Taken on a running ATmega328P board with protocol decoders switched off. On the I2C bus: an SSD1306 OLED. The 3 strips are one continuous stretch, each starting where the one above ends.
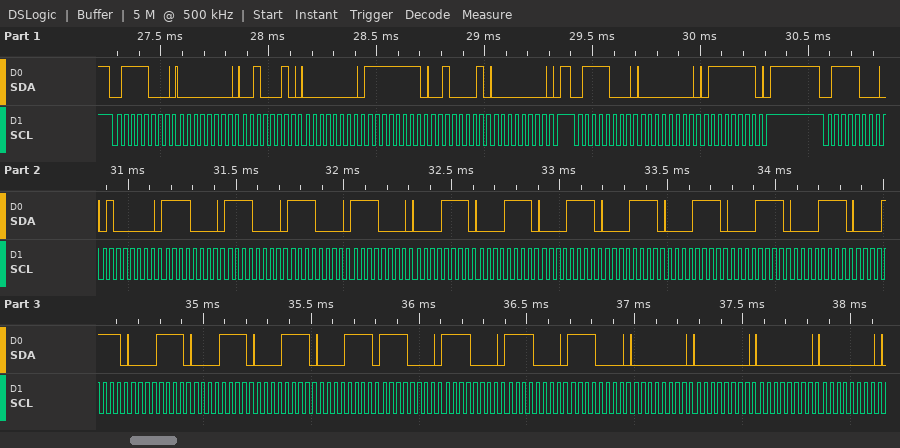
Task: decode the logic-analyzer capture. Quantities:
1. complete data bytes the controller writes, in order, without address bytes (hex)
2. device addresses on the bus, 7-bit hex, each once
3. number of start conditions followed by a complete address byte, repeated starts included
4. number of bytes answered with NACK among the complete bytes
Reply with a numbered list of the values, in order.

1. 00 22 00 FF 21 00 00 7F 40 F0 F0 F0 F0 0F 0F 0F 0F 0F 0F 0F 0F 0F 0F 0F 0F F0 F0 F0 F0 00 00 00 00
2. 0x3C
3. 3
4. 0
